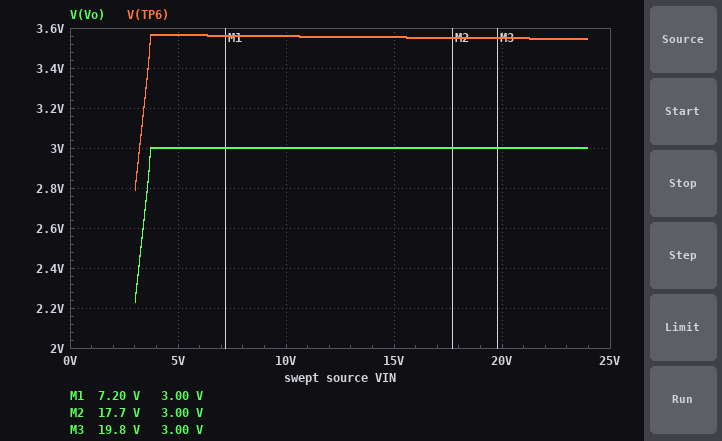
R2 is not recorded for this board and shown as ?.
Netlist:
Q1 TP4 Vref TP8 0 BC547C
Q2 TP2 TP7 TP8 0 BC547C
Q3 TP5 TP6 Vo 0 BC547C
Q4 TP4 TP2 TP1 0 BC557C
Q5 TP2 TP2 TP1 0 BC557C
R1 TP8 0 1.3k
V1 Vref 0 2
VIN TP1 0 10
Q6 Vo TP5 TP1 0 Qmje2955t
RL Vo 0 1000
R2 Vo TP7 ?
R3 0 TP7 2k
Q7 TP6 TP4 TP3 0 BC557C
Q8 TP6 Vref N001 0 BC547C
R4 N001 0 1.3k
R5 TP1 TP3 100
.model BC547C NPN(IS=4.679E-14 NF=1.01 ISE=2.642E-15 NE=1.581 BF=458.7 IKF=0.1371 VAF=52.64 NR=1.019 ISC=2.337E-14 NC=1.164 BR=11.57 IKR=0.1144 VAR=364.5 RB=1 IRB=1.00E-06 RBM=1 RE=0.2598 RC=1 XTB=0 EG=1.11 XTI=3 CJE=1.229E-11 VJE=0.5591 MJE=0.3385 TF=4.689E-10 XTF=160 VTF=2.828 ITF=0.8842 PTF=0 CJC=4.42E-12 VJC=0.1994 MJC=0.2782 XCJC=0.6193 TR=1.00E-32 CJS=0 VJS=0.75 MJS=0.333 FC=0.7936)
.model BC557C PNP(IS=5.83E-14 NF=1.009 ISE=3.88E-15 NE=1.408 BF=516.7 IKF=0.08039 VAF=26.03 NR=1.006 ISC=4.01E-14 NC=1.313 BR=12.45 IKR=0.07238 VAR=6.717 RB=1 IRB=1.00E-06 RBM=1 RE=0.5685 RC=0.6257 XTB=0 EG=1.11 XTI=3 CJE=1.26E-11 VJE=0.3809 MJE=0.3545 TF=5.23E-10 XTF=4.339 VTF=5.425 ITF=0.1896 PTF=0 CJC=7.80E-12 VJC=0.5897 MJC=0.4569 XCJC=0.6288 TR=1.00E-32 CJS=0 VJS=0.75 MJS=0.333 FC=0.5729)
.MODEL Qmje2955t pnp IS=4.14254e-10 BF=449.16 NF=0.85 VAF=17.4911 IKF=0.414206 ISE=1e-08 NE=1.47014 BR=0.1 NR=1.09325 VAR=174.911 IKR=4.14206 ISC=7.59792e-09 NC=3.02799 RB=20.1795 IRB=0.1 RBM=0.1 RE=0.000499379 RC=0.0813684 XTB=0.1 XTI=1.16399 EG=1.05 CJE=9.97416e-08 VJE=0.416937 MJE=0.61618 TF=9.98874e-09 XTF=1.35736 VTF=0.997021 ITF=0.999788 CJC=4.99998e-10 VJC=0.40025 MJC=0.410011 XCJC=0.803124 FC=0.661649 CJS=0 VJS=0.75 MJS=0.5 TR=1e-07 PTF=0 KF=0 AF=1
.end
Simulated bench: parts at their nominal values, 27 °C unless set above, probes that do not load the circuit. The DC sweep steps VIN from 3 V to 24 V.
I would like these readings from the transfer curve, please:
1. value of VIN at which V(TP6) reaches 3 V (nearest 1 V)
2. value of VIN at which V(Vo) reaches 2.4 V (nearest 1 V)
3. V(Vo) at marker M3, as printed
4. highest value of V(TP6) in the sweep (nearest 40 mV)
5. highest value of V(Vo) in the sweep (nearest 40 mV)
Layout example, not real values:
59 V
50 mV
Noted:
3 V
3 V
3.00 V
3.56 V
3.00 V
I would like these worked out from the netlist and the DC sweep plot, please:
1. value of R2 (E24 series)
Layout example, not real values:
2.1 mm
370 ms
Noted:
1 kΩ
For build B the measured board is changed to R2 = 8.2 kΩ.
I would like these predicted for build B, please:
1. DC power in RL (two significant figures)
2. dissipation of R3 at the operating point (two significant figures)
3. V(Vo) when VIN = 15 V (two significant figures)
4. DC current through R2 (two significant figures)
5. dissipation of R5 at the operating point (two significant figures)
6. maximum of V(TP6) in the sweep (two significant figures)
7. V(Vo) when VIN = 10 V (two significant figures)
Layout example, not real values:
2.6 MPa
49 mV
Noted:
85 mW
1.6 mW
10 V
900 µA
450 µW
11 V
9.2 V
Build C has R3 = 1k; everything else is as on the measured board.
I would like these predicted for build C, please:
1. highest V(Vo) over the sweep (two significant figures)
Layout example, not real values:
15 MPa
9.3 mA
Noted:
4.0 V
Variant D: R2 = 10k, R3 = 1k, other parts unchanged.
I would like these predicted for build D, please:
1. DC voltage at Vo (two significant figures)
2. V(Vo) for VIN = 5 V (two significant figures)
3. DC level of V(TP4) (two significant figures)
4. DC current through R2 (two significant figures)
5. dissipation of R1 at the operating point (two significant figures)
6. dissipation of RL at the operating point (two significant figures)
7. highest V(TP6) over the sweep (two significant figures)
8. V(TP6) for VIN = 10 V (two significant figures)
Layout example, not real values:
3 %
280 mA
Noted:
9.2 V
4.2 V
9.1 V
840 µA
1.5 mW
85 mW
23 V
9.8 V
